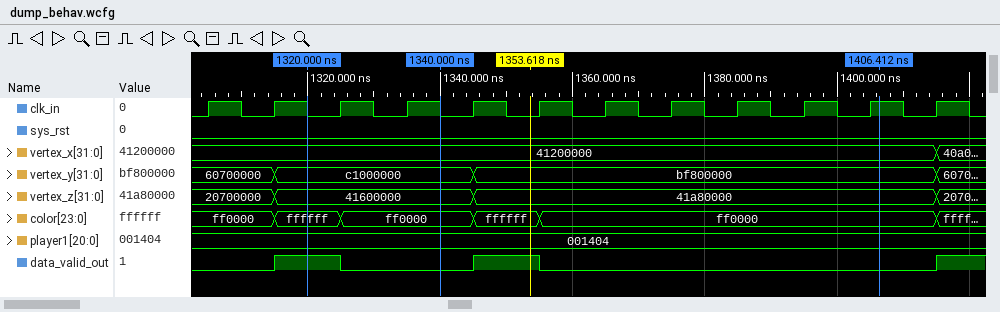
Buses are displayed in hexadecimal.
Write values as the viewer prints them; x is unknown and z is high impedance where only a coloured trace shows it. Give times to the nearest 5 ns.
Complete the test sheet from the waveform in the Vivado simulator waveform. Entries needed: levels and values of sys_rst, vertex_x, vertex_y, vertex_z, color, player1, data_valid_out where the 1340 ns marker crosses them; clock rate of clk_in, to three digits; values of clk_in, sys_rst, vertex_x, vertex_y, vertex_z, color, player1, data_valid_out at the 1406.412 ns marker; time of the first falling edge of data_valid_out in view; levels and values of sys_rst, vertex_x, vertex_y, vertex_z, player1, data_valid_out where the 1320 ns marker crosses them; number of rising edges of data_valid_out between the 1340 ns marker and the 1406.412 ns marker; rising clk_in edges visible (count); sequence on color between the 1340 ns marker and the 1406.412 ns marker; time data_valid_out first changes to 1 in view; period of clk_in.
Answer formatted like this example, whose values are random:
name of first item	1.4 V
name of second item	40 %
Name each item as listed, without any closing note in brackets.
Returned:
levels and values of sys_rst, vertex_x, vertex_y, vertex_z, color, player1, data_valid_out where the 1340 ns marker crosses them	sys_rst=0, vertex_x=41200000, vertex_y=c1000000, vertex_z=41600000, color=ff0000, player1=001404, data_valid_out=0
clock rate of clk_in, to three digits	100 MHz
values of clk_in, sys_rst, vertex_x, vertex_y, vertex_z, color, player1, data_valid_out at the 1406.412 ns marker	clk_in=1, sys_rst=0, vertex_x=41200000, vertex_y=bf800000, vertex_z=41a80000, color=ff0000, player1=001404, data_valid_out=0
time of the first falling edge of data_valid_out in view	1325 ns
levels and values of sys_rst, vertex_x, vertex_y, vertex_z, player1, data_valid_out where the 1320 ns marker crosses them	sys_rst=0, vertex_x=41200000, vertex_y=c1000000, vertex_z=41600000, player1=001404, data_valid_out=1
number of rising edges of data_valid_out between the 1340 ns marker and the 1406.412 ns marker	1
rising clk_in edges visible	12
sequence on color between the 1340 ns marker and the 1406.412 ns marker	ff0000, ffffff, ff0000
time data_valid_out first changes to 1 in view	1315 ns
period of clk_in	10 ns
